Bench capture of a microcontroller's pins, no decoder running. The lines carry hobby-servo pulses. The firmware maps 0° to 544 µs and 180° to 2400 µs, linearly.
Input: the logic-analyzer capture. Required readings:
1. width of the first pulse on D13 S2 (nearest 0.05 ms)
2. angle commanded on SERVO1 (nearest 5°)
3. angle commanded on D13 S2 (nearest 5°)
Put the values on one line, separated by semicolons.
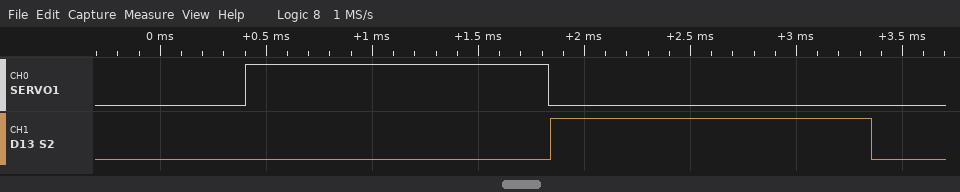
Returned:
1.50 ms; 85°; 95°
